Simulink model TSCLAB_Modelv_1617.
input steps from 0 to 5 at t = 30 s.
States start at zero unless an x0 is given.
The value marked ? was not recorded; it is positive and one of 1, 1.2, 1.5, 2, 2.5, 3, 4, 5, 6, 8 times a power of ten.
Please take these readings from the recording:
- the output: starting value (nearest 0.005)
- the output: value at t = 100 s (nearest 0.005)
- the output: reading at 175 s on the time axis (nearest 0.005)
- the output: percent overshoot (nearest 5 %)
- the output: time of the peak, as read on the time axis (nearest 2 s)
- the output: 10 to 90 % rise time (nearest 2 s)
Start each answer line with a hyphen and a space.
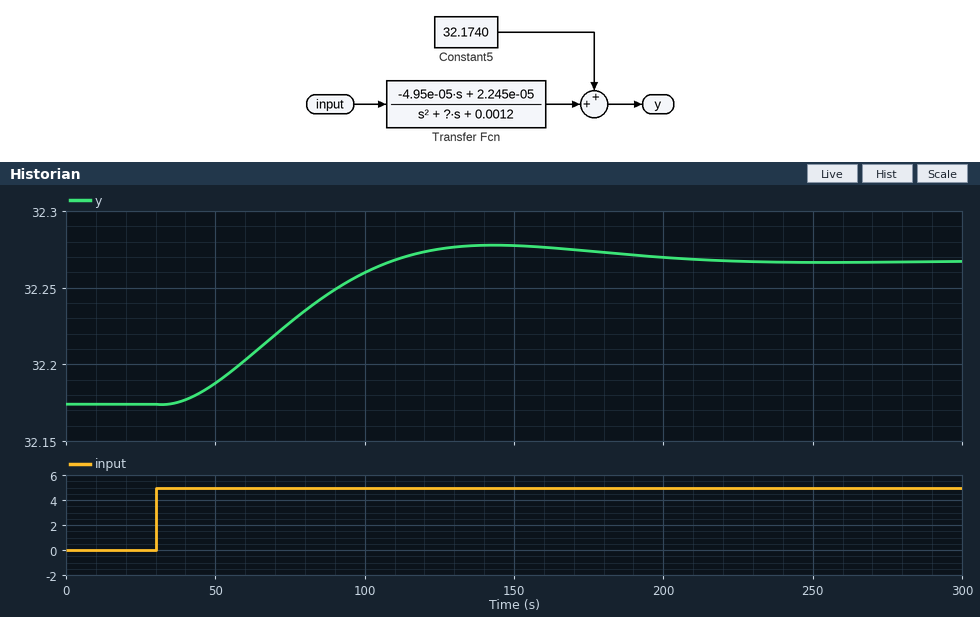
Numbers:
- 32.175
- 32.260
- 32.275
- 10 %
- 144 s
- 52 s
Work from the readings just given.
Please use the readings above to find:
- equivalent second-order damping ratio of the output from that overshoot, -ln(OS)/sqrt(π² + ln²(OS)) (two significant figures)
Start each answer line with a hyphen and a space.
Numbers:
- 0.59
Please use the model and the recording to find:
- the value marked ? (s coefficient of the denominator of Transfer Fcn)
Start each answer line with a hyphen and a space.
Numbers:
- 0.04
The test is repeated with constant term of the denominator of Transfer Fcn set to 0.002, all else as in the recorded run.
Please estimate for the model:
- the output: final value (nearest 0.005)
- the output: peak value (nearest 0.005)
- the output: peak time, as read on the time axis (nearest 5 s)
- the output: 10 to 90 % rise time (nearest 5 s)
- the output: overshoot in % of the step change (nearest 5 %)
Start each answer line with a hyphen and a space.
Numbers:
- 32.230
- 32.240
- 110 s
- 35 s
- 20 %
